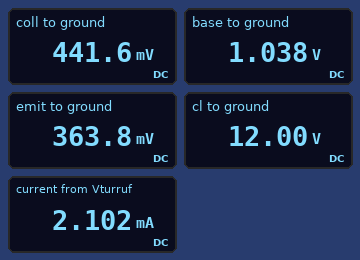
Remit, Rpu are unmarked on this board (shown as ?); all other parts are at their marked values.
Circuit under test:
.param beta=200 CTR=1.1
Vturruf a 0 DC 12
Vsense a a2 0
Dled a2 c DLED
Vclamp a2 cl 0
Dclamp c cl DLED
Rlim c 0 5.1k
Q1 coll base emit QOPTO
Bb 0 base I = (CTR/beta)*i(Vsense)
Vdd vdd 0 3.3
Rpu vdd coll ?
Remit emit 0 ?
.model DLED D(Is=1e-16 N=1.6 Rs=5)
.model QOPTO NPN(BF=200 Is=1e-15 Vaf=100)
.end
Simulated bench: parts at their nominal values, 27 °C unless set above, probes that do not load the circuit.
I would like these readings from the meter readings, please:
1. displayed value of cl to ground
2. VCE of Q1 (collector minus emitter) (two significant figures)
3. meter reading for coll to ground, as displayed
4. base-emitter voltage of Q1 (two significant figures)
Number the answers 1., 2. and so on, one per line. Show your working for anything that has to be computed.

1. 12.00 V
2. 441.6 mV - 363.8 mV = 78 mV
3. 441.6 mV
4. 1.038 V - 363.8 mV = 670 mV
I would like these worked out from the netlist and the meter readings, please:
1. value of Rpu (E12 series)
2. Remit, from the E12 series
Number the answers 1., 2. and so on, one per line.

1. 15 kΩ
2. 1.8 kΩ
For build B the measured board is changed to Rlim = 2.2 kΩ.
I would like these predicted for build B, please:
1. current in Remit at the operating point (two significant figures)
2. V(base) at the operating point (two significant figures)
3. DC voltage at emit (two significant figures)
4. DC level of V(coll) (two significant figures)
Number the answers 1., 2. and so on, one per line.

1. 220 µA
2. 1.1 V
3. 390 mV
4. 450 mV
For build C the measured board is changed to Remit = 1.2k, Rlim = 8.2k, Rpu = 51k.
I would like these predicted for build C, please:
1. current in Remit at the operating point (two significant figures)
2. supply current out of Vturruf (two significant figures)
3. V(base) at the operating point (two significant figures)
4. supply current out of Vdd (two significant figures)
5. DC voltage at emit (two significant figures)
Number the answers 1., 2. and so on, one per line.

1. 69 µA
2. 1.3 mA
3. 730 mV
4. 62 µA
5. 83 mV
